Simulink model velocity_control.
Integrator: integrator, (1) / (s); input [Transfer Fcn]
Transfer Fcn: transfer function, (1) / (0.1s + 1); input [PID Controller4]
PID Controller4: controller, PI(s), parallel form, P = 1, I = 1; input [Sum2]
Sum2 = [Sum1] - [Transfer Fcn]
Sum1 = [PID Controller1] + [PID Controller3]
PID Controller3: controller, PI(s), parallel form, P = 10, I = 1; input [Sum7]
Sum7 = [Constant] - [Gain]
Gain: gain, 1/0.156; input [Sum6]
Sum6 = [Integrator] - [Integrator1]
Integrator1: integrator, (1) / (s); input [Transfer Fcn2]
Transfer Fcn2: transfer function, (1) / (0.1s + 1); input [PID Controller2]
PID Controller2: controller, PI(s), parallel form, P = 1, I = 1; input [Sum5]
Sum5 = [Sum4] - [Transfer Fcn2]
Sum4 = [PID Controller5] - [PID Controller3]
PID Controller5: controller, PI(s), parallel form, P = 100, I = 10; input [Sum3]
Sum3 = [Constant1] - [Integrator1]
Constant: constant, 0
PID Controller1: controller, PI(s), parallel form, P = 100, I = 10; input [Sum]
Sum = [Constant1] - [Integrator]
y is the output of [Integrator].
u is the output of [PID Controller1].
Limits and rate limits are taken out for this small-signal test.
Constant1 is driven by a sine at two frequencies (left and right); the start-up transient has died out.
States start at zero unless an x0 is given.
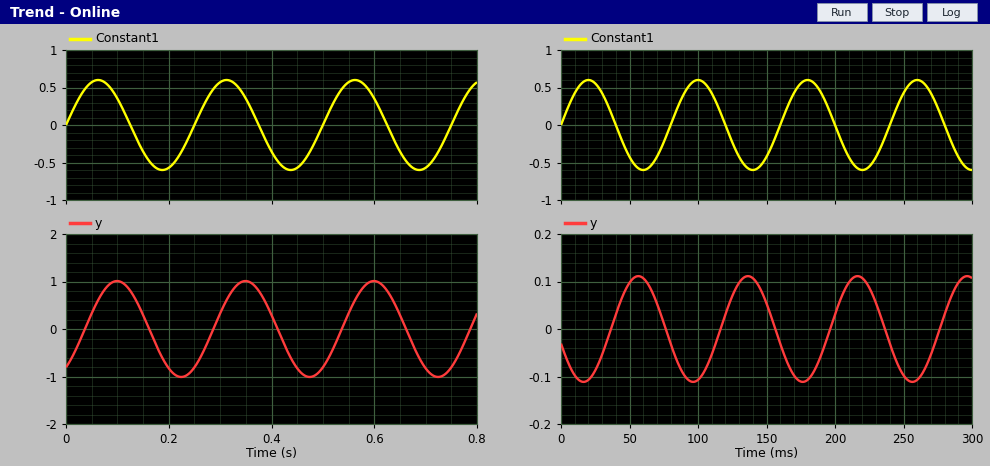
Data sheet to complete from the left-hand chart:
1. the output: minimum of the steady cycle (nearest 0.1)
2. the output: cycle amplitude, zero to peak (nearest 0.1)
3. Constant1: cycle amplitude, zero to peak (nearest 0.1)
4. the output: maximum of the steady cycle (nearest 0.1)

-1.0
1.0
0.6
1.0
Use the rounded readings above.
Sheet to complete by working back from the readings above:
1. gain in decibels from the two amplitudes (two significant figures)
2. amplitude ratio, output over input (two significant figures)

4.4 dB
1.7
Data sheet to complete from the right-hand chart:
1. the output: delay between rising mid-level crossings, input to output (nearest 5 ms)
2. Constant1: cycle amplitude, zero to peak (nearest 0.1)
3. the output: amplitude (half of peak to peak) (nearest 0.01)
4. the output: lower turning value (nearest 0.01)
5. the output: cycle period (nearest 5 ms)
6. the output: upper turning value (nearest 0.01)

35 ms
0.6
0.11
-0.11
80 ms
0.11
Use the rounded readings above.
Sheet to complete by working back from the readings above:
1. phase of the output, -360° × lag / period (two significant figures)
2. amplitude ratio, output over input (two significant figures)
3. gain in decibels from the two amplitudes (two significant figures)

-160°
0.18
-15 dB
